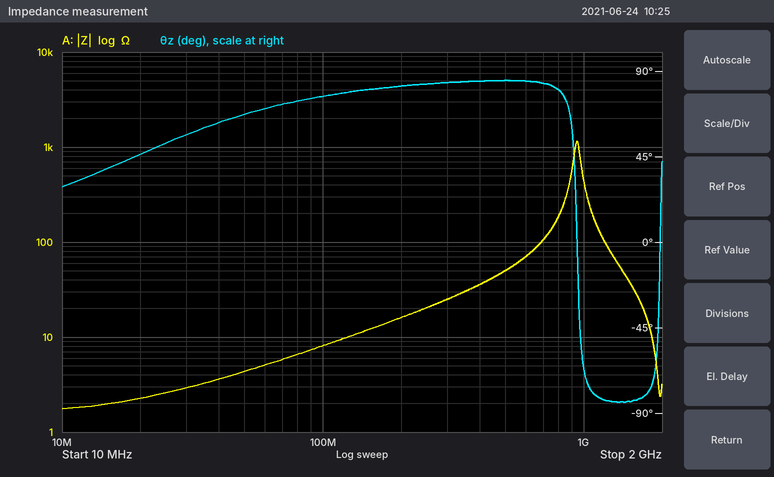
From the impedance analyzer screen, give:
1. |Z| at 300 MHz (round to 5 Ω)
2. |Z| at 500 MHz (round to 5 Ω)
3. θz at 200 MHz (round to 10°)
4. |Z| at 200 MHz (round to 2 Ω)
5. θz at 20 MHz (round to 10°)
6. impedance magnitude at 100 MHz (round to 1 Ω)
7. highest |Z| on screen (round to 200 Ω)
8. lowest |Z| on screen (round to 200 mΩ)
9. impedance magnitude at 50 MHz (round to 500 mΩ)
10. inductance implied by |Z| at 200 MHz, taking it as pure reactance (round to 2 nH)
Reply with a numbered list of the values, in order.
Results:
1. 25 Ω
2. 50 Ω
3. 80°
4. 16 Ω
5. 50°
6. 8 Ω
7. 1.2 kΩ
8. 1.8 Ω
9. 4.5 Ω
10. 12 nH
